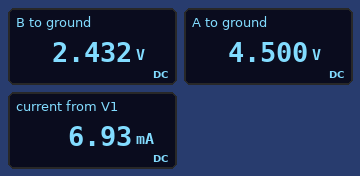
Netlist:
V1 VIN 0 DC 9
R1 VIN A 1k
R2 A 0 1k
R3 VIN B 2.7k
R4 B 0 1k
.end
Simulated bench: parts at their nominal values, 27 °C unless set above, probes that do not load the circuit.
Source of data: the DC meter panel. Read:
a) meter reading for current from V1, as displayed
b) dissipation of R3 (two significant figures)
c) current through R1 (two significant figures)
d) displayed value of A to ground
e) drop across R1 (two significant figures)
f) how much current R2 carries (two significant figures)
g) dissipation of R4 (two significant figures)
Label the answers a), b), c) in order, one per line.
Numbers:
a) 6.93 mA
b) 16 mW
c) 4.5 mA
d) 4.500 V
e) 4.5 V
f) 4.5 mA
g) 5.9 mW
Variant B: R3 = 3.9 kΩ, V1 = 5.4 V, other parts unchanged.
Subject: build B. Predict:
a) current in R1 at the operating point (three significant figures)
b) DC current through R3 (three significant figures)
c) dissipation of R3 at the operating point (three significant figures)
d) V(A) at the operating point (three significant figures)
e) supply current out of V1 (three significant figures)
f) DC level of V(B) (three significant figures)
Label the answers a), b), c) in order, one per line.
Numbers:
a) 2.70 mA
b) 1.10 mA
c) 4.74 mW
d) 2.70 V
e) 3.80 mA
f) 1.10 V
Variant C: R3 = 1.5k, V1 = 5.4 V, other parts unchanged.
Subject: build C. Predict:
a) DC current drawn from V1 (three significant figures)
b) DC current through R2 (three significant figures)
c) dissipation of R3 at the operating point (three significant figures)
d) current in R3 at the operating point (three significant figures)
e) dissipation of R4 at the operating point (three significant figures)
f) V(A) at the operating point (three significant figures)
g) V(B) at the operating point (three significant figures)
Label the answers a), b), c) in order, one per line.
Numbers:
a) 4.86 mA
b) 2.70 mA
c) 7.00 mW
d) 2.16 mA
e) 4.67 mW
f) 2.70 V
g) 2.16 V
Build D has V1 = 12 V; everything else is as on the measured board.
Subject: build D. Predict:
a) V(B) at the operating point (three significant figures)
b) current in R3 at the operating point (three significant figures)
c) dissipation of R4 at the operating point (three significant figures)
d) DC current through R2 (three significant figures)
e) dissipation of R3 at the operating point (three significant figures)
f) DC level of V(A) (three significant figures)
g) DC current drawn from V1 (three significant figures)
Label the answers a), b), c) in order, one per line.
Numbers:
a) 3.24 V
b) 3.24 mA
c) 10.5 mW
d) 6.00 mA
e) 28.4 mW
f) 6.00 V
g) 9.24 mA
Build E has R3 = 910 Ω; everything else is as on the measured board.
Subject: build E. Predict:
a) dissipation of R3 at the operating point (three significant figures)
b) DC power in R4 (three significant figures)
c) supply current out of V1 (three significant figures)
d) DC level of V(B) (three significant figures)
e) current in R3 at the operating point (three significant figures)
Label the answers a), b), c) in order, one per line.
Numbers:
a) 20.2 mW
b) 22.2 mW
c) 9.21 mA
d) 4.71 V
e) 4.71 mA
